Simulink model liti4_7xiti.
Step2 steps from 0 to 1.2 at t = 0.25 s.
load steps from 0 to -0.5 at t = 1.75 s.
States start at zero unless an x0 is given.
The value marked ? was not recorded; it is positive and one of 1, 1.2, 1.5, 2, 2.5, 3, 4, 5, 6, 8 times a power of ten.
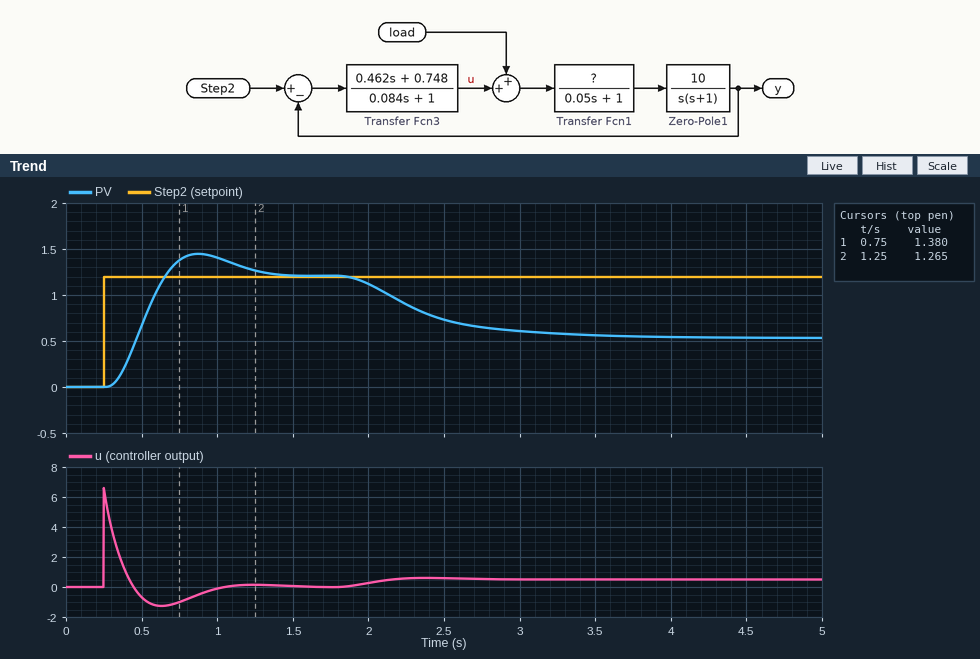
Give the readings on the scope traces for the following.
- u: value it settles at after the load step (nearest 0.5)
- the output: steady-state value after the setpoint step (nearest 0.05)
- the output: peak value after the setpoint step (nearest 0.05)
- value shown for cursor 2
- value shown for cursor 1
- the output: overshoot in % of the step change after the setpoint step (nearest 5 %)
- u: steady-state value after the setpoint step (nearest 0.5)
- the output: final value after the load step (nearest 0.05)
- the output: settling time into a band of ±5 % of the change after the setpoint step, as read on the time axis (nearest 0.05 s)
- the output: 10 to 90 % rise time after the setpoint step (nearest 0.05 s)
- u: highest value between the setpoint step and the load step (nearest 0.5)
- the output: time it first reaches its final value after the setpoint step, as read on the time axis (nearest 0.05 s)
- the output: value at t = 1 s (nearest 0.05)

0.5
1.20
1.45
1.265
1.380
20 %
0.0
0.55
1.25 s
0.25 s
6.5
0.65 s
1.40
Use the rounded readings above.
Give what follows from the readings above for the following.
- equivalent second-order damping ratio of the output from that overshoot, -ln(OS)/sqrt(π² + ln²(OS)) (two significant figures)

0.46
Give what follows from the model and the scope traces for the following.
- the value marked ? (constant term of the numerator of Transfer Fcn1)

1
